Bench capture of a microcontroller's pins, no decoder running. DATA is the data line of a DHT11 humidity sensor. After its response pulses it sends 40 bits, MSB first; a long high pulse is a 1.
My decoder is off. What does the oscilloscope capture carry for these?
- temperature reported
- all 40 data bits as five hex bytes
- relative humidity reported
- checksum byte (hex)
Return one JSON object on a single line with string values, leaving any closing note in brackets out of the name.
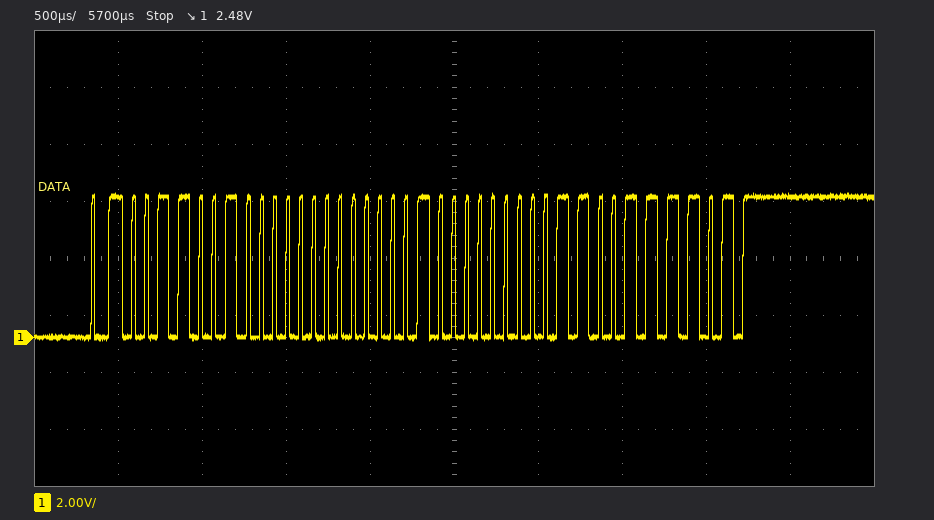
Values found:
{"temperature reported": "8.3 °C", "all 40 data bits as five hex bytes": "32 00 08 03 3D", "relative humidity reported": "50 %", "checksum byte": "0x3D"}
